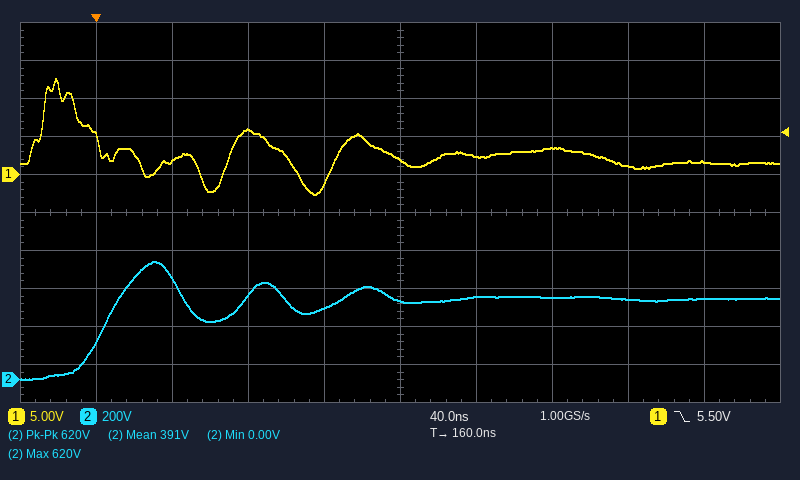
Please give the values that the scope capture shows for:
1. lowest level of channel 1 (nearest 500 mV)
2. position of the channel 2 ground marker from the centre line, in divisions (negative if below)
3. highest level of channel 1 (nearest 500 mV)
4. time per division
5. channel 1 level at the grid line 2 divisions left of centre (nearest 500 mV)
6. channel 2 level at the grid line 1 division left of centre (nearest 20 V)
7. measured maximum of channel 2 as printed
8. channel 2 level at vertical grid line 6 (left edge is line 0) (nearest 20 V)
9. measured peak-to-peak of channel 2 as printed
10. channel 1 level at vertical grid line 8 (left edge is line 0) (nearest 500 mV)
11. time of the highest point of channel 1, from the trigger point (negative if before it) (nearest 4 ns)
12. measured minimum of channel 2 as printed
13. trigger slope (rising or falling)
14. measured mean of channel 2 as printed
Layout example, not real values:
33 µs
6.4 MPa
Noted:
-2.5 V
-4.4 div
12.5 V
40 ns
6.0 V
380 V
620 V
440 V
620 V
1.0 V
-20 ns
0.00 V
falling
391 V
